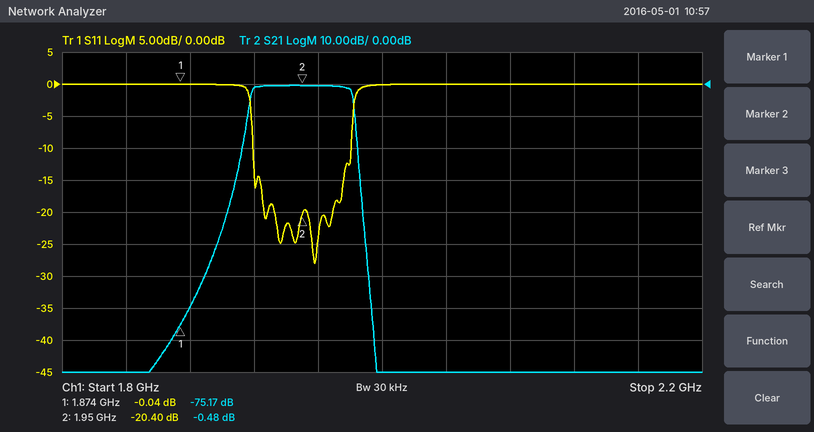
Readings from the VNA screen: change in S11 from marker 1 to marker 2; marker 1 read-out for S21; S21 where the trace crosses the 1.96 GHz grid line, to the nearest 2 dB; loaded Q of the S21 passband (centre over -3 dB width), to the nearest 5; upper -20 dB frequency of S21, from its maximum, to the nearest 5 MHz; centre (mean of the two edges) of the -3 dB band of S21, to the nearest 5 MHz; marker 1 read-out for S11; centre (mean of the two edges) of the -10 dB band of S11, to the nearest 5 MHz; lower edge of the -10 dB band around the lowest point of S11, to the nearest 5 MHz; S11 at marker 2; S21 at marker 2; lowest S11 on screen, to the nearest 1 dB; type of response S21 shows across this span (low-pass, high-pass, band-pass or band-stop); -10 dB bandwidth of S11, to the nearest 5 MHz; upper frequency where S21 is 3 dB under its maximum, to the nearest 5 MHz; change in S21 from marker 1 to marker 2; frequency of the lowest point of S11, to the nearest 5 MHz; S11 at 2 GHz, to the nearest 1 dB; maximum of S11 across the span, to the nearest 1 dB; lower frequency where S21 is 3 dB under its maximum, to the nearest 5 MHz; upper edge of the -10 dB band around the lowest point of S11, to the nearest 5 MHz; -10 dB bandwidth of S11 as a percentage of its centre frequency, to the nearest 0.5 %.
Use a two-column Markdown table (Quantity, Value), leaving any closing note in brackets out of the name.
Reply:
| Quantity | Value |
|---|---|
| change in S11 from marker 1 to marker 2 | -20.36 dB |
| marker 1 read-out for S21 | -75.17 dB |
| S21 where the trace crosses the 1.96 GHz grid line, to the nearest 2 dB | 0 dB |
| loaded Q of the S21 passband (centre over -3 dB width), to the nearest 5 | 30 |
| upper -20 dB frequency of S21, from its maximum, to the nearest 5 MHz | 1.985 GHz |
| centre (mean of the two edges) of the -3 dB band of S21, to the nearest 5 MHz | 1.950 GHz |
| marker 1 read-out for S11 | -0.04 dB |
| centre (mean of the two edges) of the -10 dB band of S11, to the nearest 5 MHz | 1.950 GHz |
| lower edge of the -10 dB band around the lowest point of S11, to the nearest 5 MHz | 1.920 GHz |
| S11 at marker 2 | -20.40 dB |
| S21 at marker 2 | -0.48 dB |
| lowest S11 on screen, to the nearest 1 dB | -28 dB |
| type of response S21 shows across this span | band-pass |
| -10 dB bandwidth of S11, to the nearest 5 MHz | 60 MHz |
| upper frequency where S21 is 3 dB under its maximum, to the nearest 5 MHz | 1.980 GHz |
| change in S21 from marker 1 to marker 2 | 74.69 dB |
| frequency of the lowest point of S11, to the nearest 5 MHz | 1.960 GHz |
| S11 at 2 GHz, to the nearest 1 dB | 0 dB |
| maximum of S11 across the span, to the nearest 1 dB | 0 dB |
| lower frequency where S21 is 3 dB under its maximum, to the nearest 5 MHz | 1.920 GHz |
| upper edge of the -10 dB band around the lowest point of S11, to the nearest 5 MHz | 1.980 GHz |
| -10 dB bandwidth of S11 as a percentage of its centre frequency, to the nearest 0.5 % | 3.0 % |
